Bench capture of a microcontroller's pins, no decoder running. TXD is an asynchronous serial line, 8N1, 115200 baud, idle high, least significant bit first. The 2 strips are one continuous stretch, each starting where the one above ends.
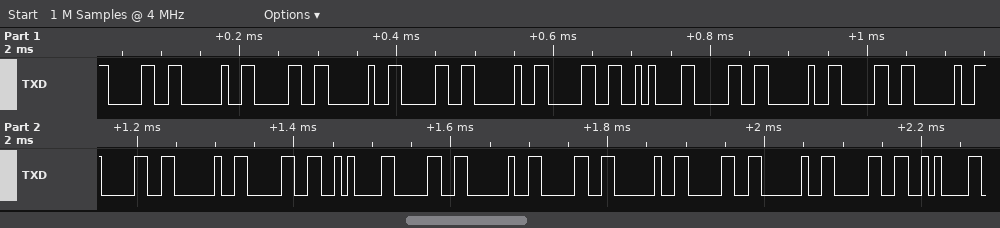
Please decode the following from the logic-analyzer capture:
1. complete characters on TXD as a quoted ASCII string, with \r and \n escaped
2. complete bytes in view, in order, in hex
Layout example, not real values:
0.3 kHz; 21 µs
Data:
"0 0 0 0\n0 0 0 0\n0 0 0 0\n"; 30 20 30 20 30 20 30 0A 30 20 30 20 30 20 30 0A 30 20 30 20 30 20 30 0A
